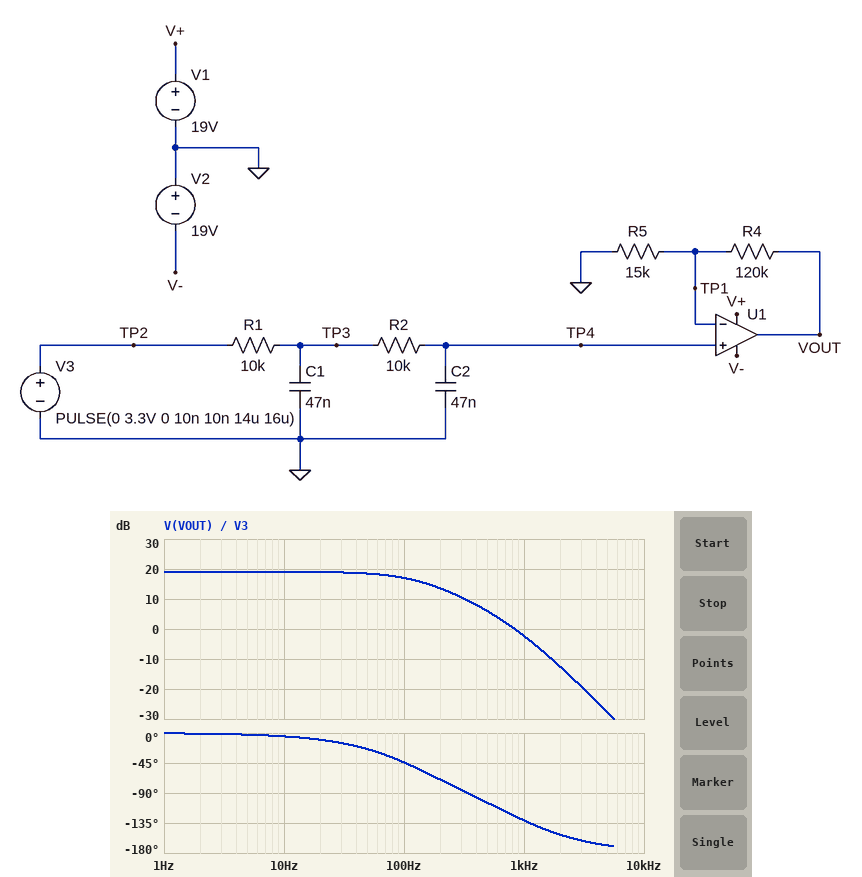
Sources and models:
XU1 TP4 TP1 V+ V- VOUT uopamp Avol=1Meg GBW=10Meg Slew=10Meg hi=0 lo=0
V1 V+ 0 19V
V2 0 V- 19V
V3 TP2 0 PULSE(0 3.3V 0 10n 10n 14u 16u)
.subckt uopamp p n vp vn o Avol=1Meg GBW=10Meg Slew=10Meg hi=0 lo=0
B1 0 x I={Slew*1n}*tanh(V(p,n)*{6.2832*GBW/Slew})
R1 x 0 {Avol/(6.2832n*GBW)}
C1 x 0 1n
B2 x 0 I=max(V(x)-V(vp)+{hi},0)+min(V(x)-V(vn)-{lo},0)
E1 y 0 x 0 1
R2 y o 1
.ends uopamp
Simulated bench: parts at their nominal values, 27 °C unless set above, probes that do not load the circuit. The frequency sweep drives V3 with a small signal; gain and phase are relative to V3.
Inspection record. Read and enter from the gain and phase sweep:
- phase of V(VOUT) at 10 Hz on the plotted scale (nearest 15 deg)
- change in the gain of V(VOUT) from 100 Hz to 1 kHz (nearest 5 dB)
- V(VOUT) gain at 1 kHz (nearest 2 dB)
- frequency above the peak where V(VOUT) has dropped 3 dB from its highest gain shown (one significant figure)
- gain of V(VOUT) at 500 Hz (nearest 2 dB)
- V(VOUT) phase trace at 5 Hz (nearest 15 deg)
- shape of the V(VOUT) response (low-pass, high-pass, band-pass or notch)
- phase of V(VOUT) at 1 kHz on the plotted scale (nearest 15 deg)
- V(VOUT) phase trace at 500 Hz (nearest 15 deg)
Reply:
0 deg
-20 dB
-2 dB
100 Hz
6 dB
0 deg
low-pass
-135 deg
-105 deg
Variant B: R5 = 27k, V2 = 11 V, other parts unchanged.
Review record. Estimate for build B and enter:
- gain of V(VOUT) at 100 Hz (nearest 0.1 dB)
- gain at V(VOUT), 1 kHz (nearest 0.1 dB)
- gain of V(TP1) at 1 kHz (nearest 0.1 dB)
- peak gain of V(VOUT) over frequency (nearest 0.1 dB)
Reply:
12.6 dB
-6.7 dB
-21.4 dB
14.7 dB
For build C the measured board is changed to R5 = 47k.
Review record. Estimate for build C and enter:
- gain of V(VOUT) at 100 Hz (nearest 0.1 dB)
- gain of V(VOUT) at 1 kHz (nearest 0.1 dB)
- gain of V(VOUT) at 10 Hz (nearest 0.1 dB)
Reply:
8.9 dB
-10.4 dB
11.0 dB
